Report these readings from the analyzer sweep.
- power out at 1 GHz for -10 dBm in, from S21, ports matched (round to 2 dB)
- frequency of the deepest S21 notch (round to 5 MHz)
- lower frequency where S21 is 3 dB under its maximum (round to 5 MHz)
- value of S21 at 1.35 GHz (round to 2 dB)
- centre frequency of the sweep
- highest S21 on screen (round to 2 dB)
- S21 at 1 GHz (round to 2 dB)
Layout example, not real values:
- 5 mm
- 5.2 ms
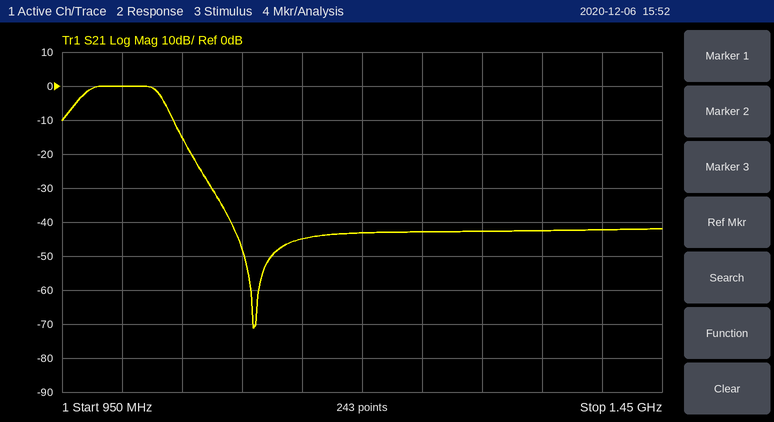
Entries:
- -10 dBm
- 1.110 GHz
- 965 MHz
- -42 dB
- 1.2 GHz
- 0 dB
- 0 dB
